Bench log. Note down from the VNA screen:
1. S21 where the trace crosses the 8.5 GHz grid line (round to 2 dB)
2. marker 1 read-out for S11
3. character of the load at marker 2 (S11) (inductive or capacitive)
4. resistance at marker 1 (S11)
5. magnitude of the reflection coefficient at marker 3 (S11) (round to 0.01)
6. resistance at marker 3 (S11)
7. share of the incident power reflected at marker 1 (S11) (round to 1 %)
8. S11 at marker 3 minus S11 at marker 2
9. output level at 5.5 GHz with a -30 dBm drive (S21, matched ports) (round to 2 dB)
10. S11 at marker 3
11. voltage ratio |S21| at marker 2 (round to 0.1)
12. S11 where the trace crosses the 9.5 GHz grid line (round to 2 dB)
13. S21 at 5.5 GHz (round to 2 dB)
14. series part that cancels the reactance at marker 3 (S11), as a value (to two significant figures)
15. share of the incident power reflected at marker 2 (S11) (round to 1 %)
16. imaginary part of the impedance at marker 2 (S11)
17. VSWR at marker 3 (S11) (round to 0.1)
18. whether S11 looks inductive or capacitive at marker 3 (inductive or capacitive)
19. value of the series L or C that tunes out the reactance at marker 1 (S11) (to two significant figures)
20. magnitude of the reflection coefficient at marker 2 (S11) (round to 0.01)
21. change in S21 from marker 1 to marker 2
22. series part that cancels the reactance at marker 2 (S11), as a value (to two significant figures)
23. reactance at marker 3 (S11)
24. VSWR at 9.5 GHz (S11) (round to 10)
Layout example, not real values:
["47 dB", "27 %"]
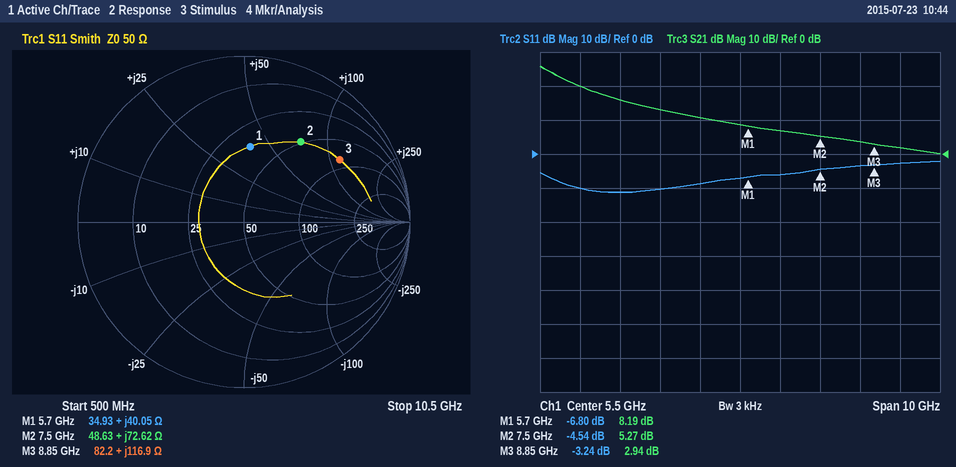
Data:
["4 dB", "-6.80 dB", "inductive", "34.93 Ω", "0.69", "82.2 Ω", "21 %", "1.30 dB", "-22 dBm", "-3.24 dB", "1.8", "-2 dB", "8 dB", "150 fF", "35 %", "+72.62 Ω", "5.4", "inductive", "700 fF", "0.59", "-2.92 dB", "290 fF", "+116.9 Ω", "10"]
